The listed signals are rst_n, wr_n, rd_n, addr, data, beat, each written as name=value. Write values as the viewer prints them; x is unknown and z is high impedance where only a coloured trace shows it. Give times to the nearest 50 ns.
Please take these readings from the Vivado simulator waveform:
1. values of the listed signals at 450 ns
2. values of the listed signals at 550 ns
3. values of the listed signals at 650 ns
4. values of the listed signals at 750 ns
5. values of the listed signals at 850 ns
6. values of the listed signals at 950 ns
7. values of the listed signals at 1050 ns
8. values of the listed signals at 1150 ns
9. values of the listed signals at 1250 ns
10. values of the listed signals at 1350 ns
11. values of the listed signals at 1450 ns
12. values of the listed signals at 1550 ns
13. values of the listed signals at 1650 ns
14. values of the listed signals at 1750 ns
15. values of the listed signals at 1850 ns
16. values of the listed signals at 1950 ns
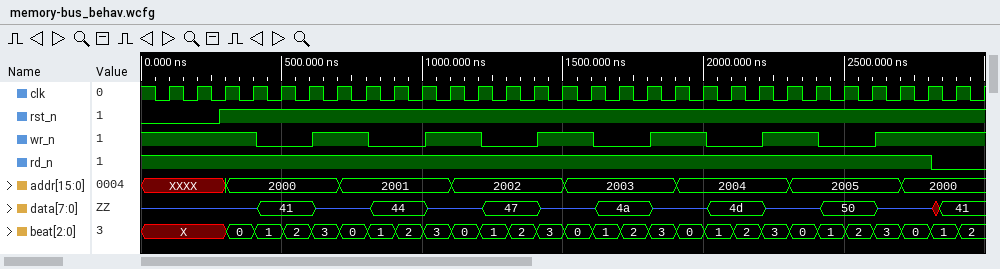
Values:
rst_n=1, wr_n=0, rd_n=1, addr=2000, data=41, beat=1
rst_n=1, wr_n=0, rd_n=1, addr=2000, data=41, beat=2
rst_n=1, wr_n=1, rd_n=1, addr=2000, data=z, beat=3
rst_n=1, wr_n=1, rd_n=1, addr=2001, data=z, beat=0
rst_n=1, wr_n=0, rd_n=1, addr=2001, data=44, beat=1
rst_n=1, wr_n=0, rd_n=1, addr=2001, data=44, beat=2
rst_n=1, wr_n=1, rd_n=1, addr=2001, data=z, beat=3
rst_n=1, wr_n=1, rd_n=1, addr=2002, data=z, beat=0
rst_n=1, wr_n=0, rd_n=1, addr=2002, data=47, beat=1
rst_n=1, wr_n=0, rd_n=1, addr=2002, data=47, beat=2
rst_n=1, wr_n=1, rd_n=1, addr=2002, data=z, beat=3
rst_n=1, wr_n=1, rd_n=1, addr=2003, data=z, beat=0
rst_n=1, wr_n=0, rd_n=1, addr=2003, data=4a, beat=1
rst_n=1, wr_n=0, rd_n=1, addr=2003, data=4a, beat=2
rst_n=1, wr_n=1, rd_n=1, addr=2003, data=z, beat=3
rst_n=1, wr_n=1, rd_n=1, addr=2004, data=z, beat=0
